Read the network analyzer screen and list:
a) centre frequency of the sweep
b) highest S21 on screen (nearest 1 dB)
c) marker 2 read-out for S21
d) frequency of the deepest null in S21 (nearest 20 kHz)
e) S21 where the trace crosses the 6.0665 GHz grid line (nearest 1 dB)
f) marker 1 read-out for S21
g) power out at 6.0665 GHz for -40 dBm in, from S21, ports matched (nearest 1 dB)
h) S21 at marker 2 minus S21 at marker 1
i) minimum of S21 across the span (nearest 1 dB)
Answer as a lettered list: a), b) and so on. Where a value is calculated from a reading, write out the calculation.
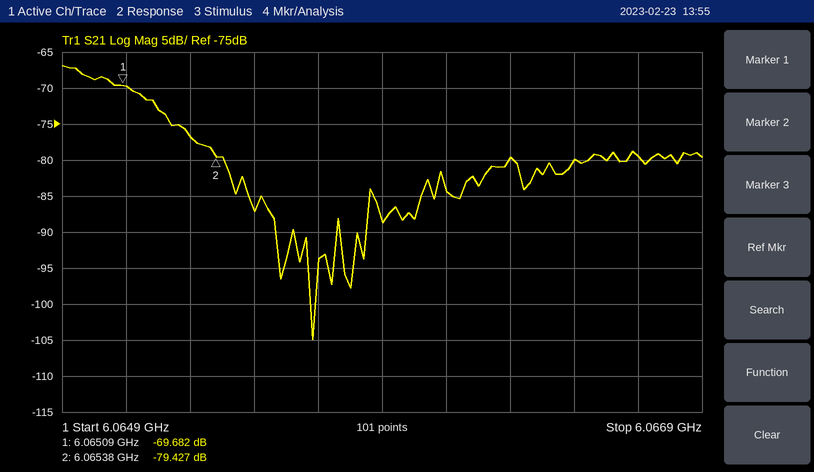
a) 6.0659 GHz
b) -67 dB
c) -79.427 dB
d) 6.06568 GHz
e) -80 dB
f) -69.682 dB
g) -40 dBm + (-80 dB) = -120 dBm
h) -79.427 − (-69.682) = -9.745 dB
i) -105 dB
